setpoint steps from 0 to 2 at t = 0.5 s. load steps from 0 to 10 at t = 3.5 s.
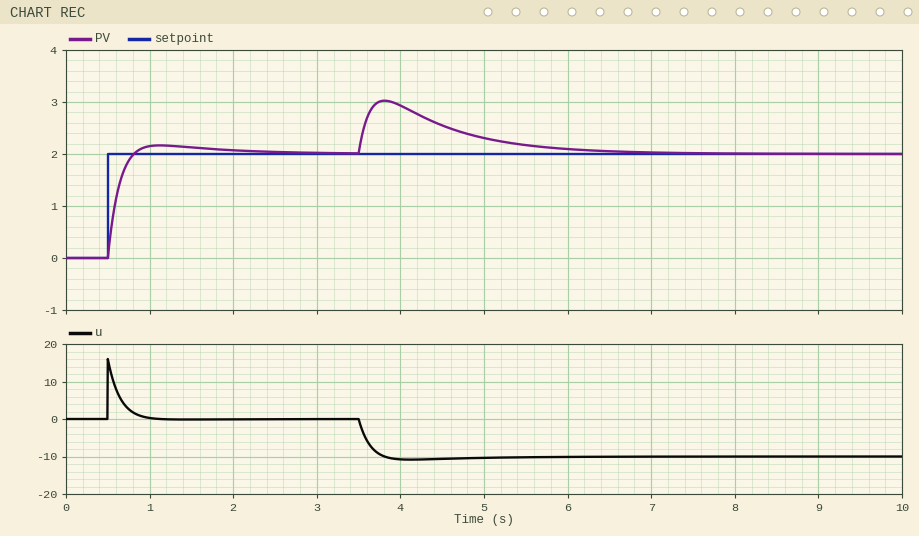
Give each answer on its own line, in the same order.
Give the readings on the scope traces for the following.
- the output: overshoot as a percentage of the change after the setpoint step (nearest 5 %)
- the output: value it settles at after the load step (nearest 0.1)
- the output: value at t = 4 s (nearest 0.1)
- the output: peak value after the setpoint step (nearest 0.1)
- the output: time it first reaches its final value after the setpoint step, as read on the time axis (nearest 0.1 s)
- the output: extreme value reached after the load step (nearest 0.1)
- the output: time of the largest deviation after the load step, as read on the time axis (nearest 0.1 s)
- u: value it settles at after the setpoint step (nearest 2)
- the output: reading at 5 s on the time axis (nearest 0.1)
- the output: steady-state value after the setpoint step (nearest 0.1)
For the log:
10 %
2.0
2.9
2.2
0.8 s
3.0
3.8 s
0
2.3
2.0
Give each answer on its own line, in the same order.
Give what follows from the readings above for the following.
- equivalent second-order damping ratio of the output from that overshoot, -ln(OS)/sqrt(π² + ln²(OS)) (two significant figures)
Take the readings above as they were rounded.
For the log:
0.59
